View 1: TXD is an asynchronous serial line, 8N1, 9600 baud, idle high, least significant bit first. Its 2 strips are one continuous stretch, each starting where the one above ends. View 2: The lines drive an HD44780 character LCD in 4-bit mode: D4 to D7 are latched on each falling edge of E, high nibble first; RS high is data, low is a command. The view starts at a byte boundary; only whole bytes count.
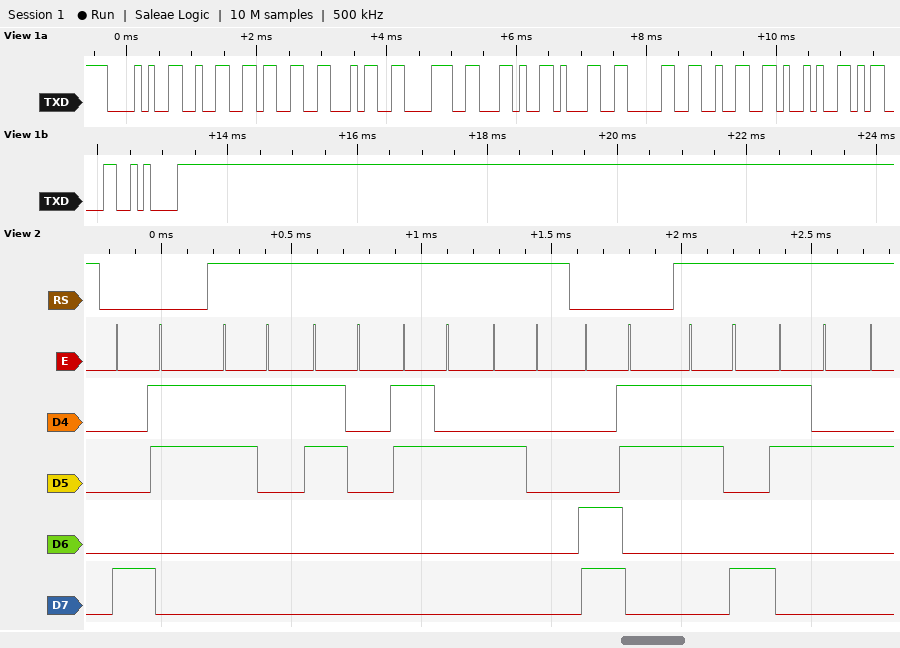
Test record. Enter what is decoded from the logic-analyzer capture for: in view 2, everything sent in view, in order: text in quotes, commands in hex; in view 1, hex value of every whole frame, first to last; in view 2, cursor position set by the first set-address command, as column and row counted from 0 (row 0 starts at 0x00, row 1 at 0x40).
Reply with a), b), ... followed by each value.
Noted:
a) 0x83 "102 " 0xC3 "92"
b) 28 32 33 34 38 2C 31 30 32 29 0D 0A
c) column 3, row 0
